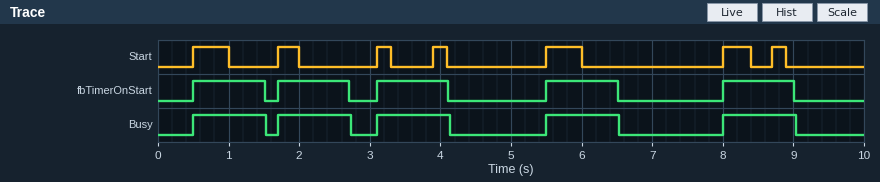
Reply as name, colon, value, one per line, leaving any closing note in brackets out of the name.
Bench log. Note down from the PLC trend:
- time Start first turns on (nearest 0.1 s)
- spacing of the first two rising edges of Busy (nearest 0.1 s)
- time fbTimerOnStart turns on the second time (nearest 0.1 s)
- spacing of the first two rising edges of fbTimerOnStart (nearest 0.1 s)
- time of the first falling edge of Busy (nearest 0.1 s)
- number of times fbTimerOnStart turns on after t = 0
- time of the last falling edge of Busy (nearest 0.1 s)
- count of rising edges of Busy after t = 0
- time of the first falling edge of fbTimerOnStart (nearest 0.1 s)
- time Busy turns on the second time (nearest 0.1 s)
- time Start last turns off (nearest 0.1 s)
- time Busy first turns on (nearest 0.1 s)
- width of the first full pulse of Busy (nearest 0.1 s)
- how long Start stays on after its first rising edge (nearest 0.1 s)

time Start first turns on: 0.5 s
spacing of the first two rising edges of Busy: 1.2 s
time fbTimerOnStart turns on the second time: 1.7 s
spacing of the first two rising edges of fbTimerOnStart: 1.2 s
time of the first falling edge of Busy: 1.5 s
number of times fbTimerOnStart turns on after t = 0: 5
time of the last falling edge of Busy: 9.0 s
count of rising edges of Busy after t = 0: 5
time of the first falling edge of fbTimerOnStart: 1.5 s
time Busy turns on the second time: 1.7 s
time Start last turns off: 8.9 s
time Busy first turns on: 0.5 s
width of the first full pulse of Busy: 1.0 s
how long Start stays on after its first rising edge: 0.5 s
